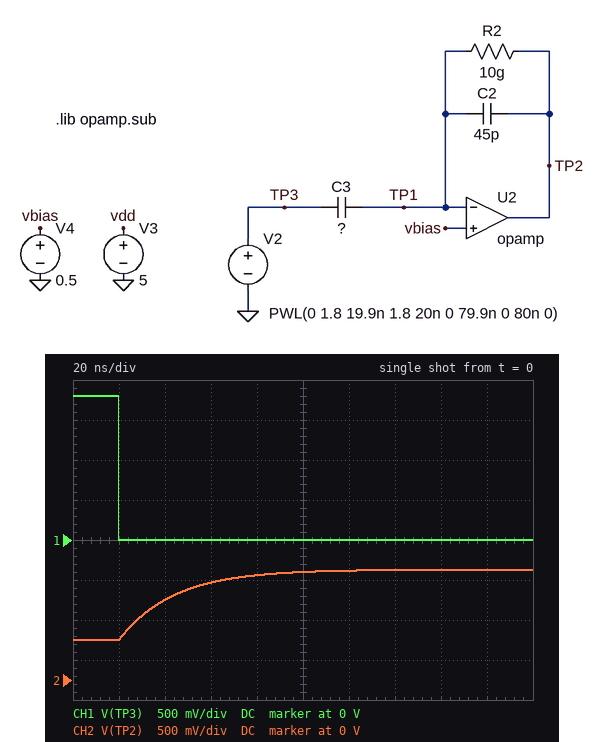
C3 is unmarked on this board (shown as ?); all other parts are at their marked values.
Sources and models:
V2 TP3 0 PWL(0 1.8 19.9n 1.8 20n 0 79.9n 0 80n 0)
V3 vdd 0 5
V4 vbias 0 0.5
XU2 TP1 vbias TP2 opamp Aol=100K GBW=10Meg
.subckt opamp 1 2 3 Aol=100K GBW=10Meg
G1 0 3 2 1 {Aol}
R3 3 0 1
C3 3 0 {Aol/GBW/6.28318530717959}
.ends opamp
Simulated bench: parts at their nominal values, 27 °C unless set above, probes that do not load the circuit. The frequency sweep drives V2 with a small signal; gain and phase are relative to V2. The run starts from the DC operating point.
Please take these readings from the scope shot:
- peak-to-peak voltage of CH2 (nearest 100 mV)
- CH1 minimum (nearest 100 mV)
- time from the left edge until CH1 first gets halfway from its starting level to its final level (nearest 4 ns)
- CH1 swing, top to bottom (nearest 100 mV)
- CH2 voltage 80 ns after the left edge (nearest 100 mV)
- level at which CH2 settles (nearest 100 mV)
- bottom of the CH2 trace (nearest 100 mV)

900 mV
0 V
20 ns
1.8 V
1.3 V
1.4 V
500 mV
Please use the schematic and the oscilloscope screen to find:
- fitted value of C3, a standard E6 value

22 pF
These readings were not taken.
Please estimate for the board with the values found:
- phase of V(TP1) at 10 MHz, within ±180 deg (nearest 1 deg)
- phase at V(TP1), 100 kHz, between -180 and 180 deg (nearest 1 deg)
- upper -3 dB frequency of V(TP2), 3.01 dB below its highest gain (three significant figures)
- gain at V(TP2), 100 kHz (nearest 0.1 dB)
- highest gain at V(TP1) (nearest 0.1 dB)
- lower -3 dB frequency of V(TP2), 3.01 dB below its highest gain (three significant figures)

34 deg
89 deg
6.72 MHz
-6.2 dB
-9.7 dB
354 mHz
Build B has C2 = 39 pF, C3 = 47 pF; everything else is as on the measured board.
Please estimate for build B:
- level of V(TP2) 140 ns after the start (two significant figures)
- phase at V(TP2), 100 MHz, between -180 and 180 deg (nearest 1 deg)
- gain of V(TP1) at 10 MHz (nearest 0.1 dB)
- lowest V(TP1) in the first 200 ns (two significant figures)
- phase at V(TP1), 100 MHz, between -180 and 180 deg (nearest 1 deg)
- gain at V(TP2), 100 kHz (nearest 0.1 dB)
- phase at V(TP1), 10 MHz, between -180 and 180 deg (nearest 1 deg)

2.6 V
93 deg
-6.1 dB
-480 mV
3 deg
1.6 dB
24 deg
